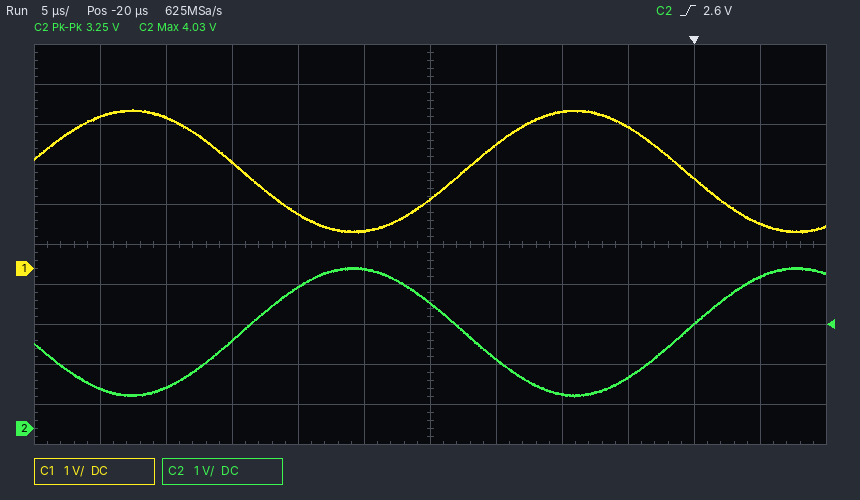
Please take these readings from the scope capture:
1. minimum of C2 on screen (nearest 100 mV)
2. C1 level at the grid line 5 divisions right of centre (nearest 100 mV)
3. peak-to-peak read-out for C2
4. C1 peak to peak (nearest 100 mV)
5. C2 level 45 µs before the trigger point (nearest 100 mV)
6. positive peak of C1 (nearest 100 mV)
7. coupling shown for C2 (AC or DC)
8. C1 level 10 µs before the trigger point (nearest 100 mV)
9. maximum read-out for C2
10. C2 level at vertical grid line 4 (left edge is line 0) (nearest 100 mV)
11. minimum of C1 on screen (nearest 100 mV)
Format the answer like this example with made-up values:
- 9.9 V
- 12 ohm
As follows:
- 800 mV
- 1.1 V
- 3.25 V
- 3.1 V
- 1.0 V
- 4.0 V
- DC
- 3.9 V
- 4.03 V
- 3.5 V
- 900 mV
